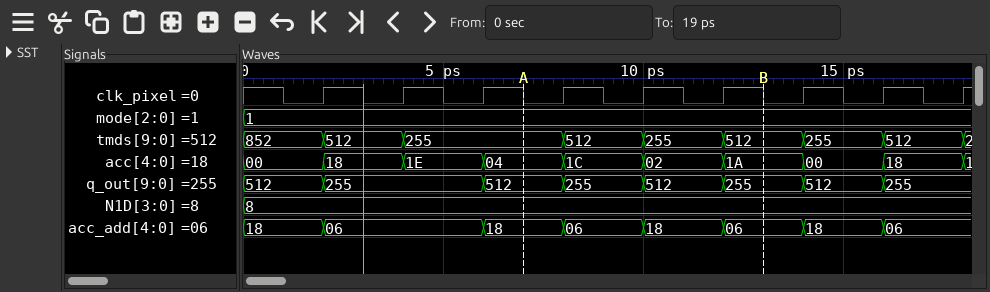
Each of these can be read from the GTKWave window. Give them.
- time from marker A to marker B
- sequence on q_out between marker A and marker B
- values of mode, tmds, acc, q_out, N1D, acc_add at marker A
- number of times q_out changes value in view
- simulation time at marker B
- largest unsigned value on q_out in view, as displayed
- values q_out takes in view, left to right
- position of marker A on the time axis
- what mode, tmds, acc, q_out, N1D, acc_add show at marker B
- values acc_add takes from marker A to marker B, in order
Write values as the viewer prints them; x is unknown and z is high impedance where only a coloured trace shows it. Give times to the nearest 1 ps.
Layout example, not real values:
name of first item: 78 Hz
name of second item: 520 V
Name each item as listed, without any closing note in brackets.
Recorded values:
time from marker A to marker B: 6 ps
sequence on q_out between marker A and marker B: 512, 255, 512, 255
values of mode, tmds, acc, q_out, N1D, acc_add at marker A: mode=1, tmds=255, acc=04, q_out=512, N1D=8, acc_add=18
number of times q_out changes value in view: 7
simulation time at marker B: 13 ps
largest unsigned value on q_out in view, as displayed: 512
values q_out takes in view, left to right: 512, 255, 512, 255, 512, 255, 512, 255
position of marker A on the time axis: 7 ps
what mode, tmds, acc, q_out, N1D, acc_add show at marker B: mode=1, tmds=512, acc=1A, q_out=255, N1D=8, acc_add=06
values acc_add takes from marker A to marker B, in order: 18, 06, 18, 06
